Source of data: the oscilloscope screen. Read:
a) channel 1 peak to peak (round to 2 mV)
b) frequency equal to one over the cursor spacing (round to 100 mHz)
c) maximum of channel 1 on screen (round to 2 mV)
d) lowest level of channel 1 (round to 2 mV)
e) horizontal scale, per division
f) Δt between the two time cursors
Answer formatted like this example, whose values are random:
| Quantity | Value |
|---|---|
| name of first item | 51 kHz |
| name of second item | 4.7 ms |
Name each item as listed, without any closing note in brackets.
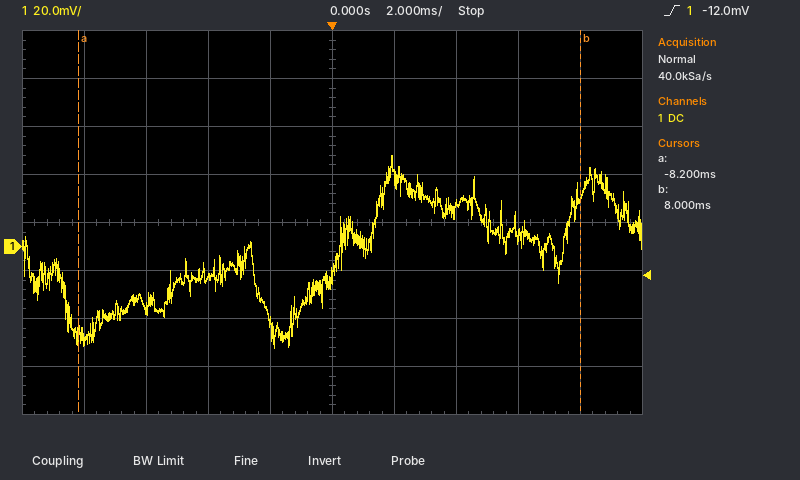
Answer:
| Quantity | Value |
|---|---|
| channel 1 peak to peak | 80 mV |
| frequency equal to one over the cursor spacing | 61.7 Hz |
| maximum of channel 1 on screen | 38 mV |
| lowest level of channel 1 | -42 mV |
| horizontal scale, per division | 2 ms |
| Δt between the two time cursors | 16.2 ms |
